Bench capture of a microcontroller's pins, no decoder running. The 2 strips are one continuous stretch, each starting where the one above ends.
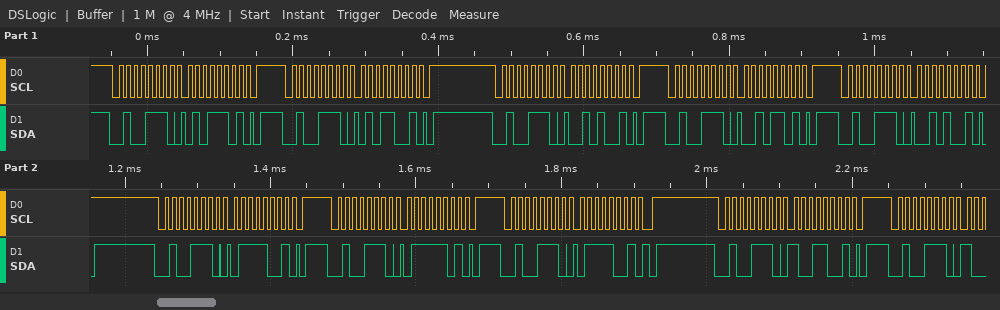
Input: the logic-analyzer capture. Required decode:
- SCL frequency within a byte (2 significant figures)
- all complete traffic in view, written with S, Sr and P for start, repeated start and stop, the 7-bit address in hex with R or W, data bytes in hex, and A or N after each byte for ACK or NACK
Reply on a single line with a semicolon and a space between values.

100 kHz; S 27W A 5D A P S 27W A 59 A P S 27W A 29 A P S 27W A 2D A P S 27W A 29 A P S 27W A 79 A P S 27W A 7D A P S 27W A 79 A P S 27W A 99 A P S 27W A
